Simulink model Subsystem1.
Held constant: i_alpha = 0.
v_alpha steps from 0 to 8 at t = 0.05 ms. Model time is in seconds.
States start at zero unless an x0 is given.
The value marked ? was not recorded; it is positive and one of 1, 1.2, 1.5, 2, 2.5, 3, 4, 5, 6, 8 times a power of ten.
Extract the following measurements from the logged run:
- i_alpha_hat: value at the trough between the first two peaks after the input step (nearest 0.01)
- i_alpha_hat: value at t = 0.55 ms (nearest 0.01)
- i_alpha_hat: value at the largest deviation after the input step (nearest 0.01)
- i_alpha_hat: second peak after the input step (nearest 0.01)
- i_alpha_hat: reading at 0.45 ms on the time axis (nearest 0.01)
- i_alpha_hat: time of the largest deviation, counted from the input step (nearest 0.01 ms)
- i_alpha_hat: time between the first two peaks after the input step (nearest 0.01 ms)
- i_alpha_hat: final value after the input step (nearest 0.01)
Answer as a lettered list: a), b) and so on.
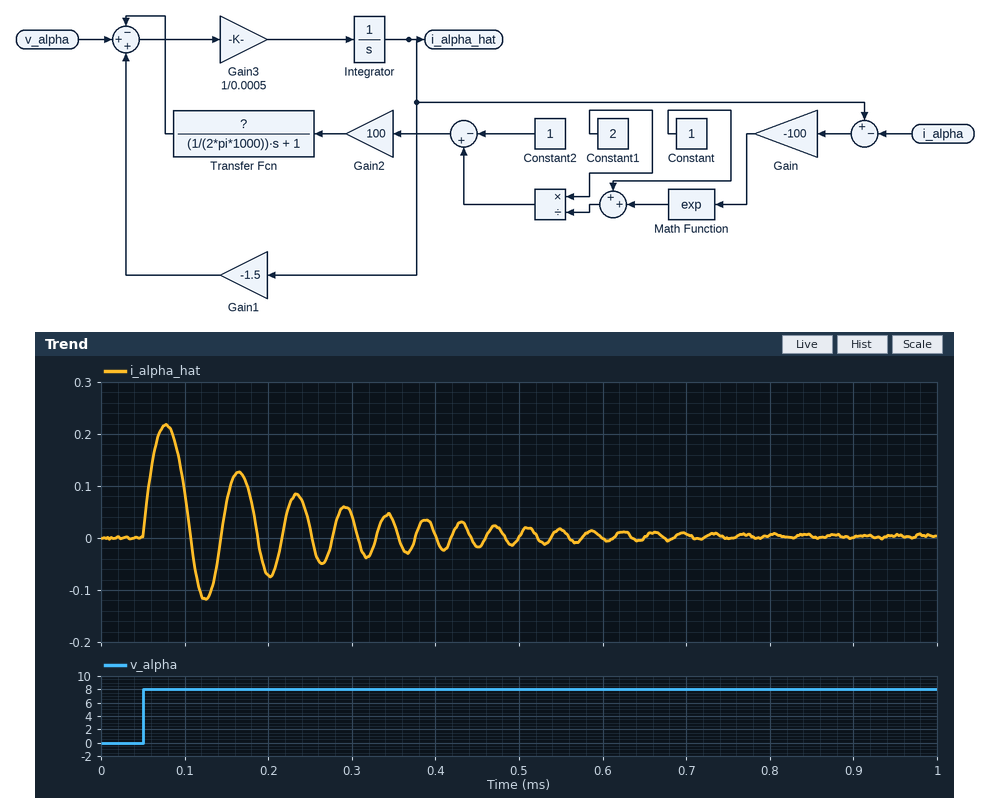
a) -0.12
b) 0.02
c) 0.22
d) 0.13
e) -0.02
f) 0.03 ms
g) 0.09 ms
h) 0.00
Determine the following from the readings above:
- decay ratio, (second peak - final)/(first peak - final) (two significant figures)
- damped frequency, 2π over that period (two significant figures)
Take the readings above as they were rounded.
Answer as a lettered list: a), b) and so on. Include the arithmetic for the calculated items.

a) (0.13 - 0) / (0.22 - 0) = 0.59
b) 2π / 0.09 = 70 rad/ms
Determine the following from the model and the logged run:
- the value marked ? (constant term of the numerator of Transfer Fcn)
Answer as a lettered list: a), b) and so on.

a) 0.5
